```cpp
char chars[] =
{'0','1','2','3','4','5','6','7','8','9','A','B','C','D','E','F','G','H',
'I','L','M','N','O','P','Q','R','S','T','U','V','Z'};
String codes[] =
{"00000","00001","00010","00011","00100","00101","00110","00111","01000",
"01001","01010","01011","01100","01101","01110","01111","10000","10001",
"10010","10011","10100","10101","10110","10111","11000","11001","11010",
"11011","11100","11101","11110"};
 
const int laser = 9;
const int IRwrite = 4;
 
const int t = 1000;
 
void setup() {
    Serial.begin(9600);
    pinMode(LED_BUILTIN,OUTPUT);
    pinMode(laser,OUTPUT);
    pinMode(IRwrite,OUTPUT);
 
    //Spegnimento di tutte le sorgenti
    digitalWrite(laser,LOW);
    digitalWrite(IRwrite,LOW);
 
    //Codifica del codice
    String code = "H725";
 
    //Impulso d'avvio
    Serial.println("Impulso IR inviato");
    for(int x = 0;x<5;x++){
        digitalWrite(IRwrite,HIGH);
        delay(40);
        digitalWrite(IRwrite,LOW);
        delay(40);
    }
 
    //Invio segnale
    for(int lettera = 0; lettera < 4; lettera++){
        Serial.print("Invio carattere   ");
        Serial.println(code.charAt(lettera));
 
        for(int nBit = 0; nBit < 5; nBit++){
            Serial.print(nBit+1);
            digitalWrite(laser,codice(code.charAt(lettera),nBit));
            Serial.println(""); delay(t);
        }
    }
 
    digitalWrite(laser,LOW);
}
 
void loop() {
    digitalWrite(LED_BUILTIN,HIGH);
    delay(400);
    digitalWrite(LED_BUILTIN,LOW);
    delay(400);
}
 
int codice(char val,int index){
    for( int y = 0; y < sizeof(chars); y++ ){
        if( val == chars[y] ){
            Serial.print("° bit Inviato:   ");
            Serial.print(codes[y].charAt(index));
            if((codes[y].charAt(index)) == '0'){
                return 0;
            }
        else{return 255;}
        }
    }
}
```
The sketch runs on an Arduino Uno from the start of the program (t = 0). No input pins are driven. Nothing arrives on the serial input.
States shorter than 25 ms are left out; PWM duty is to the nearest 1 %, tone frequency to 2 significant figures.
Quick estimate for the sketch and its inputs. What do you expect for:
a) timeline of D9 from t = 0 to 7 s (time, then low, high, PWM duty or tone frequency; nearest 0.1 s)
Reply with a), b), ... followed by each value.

a) 0 s low; 0.4 s high; 1.4 s low; 4.4 s high; 5.4 s low
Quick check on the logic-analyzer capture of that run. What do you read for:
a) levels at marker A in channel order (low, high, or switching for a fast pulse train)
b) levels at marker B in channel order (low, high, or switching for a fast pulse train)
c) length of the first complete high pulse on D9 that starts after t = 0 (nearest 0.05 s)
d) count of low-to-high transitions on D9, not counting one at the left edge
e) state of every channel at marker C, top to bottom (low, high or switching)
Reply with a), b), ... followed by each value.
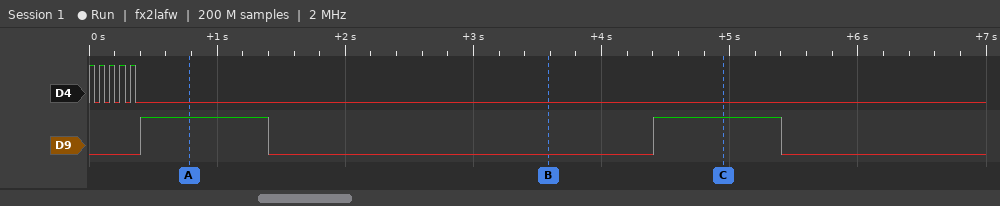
a) D4 low, D9 high
b) D4 low, D9 low
c) 1.00 s
d) 2
e) D4 low, D9 high
